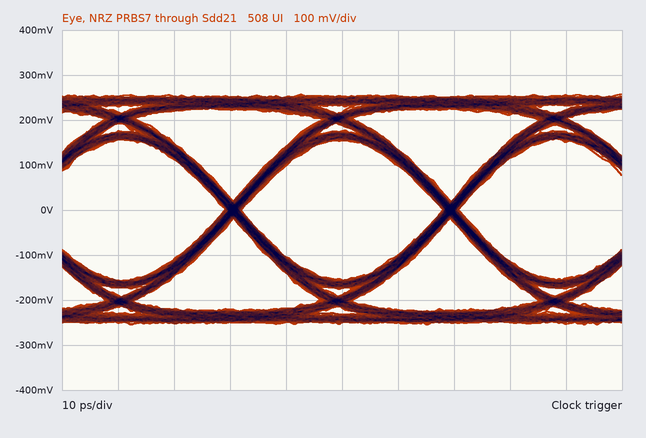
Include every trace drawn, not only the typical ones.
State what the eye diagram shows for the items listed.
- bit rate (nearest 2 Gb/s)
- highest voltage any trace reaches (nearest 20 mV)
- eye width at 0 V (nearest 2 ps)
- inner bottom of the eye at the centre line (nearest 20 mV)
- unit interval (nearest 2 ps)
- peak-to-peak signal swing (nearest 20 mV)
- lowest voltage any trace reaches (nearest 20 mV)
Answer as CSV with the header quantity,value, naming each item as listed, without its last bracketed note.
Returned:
quantity,value
bit rate,26 Gb/s
highest voltage any trace reaches,260 mV
eye width at 0 V,36 ps
inner bottom of the eye at the centre line,-160 mV
unit interval,38 ps
peak-to-peak signal swing,520 mV
lowest voltage any trace reaches,-260 mV
